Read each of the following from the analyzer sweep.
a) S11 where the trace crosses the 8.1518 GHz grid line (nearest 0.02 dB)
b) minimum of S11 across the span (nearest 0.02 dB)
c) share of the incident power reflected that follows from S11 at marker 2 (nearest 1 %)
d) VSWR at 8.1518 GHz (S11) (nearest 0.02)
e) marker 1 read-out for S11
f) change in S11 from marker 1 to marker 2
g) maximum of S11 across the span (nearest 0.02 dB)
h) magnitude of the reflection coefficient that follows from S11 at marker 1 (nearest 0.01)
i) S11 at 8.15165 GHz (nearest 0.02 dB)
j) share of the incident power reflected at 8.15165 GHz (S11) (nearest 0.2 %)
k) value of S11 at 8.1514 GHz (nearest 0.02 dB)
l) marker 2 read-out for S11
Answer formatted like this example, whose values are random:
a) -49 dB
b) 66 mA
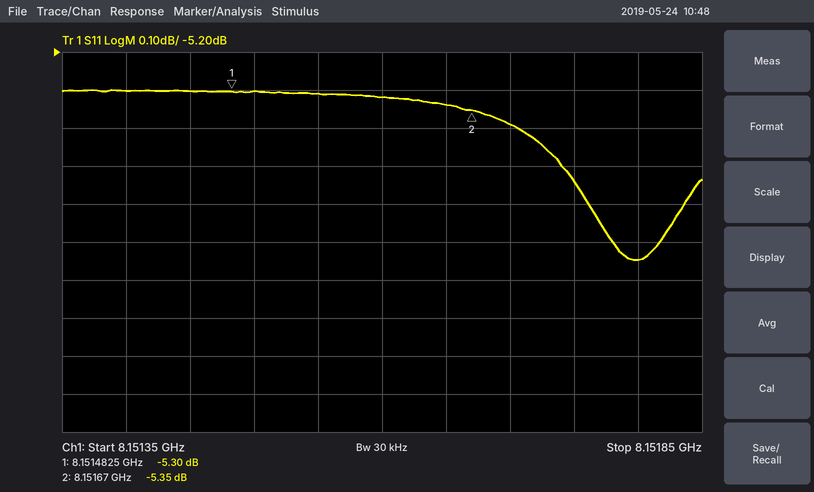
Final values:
a) -5.74 dB
b) -5.74 dB
c) 29 %
d) 3.14
e) -5.30 dB
f) -0.05 dB
g) -5.30 dB
h) 0.54
i) -5.34 dB
j) 29.2 %
k) -5.30 dB
l) -5.35 dB
